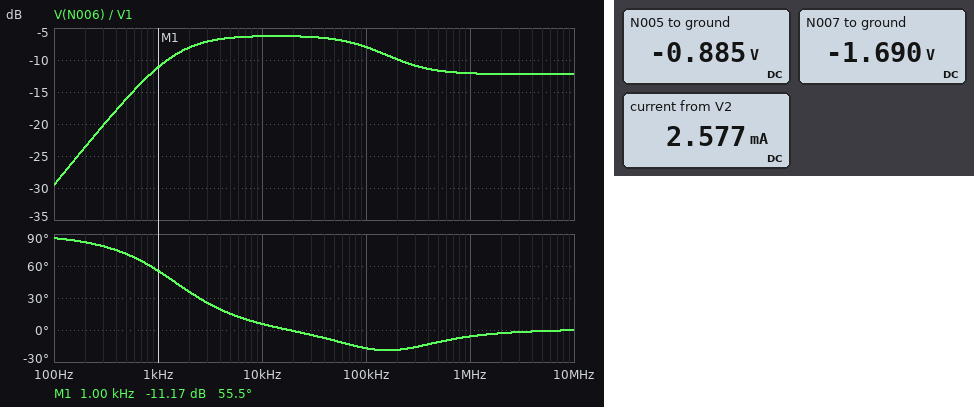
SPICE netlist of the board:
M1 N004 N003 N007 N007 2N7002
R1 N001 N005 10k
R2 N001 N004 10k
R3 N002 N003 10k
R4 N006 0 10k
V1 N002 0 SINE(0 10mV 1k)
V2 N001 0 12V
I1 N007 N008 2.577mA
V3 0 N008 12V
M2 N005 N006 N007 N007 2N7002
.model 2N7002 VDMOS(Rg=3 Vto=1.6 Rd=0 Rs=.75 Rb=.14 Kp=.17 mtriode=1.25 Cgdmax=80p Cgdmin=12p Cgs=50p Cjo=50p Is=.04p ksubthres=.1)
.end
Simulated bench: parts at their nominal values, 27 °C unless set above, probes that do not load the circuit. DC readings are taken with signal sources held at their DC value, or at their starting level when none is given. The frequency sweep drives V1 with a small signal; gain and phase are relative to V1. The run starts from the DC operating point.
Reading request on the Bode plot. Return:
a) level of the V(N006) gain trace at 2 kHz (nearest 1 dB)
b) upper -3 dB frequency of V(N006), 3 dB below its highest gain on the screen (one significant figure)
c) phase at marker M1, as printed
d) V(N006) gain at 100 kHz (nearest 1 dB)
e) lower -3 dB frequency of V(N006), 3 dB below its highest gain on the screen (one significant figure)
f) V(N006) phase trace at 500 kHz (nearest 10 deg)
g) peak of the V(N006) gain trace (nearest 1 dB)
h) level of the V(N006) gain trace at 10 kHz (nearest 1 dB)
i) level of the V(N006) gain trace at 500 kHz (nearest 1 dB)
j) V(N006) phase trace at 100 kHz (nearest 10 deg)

-8 dB
200 kHz
55.5 deg
-8 dB
1 kHz
-10 deg
-6 dB
-6 dB
-12 dB
-20 deg
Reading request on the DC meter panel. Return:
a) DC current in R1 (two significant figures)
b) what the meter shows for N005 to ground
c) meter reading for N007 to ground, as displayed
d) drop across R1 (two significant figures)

1.3 mA
-0.885 V
-1.690 V
13 V
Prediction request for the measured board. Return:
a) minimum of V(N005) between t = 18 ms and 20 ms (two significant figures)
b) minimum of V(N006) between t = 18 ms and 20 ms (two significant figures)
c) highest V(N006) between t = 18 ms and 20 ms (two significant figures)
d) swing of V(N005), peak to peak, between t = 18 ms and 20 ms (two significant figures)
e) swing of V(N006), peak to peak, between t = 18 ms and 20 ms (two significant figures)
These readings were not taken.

-1.5 V
-2.8 mV
2.8 mV
1.2 V
5.5 mV
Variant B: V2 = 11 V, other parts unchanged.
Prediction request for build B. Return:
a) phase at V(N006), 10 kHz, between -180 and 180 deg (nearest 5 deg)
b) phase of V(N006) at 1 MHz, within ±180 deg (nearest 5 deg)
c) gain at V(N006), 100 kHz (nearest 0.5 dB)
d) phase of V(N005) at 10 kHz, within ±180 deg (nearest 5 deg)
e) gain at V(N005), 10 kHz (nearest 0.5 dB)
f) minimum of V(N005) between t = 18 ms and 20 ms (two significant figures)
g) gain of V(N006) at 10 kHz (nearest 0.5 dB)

125 deg
10 deg
-17.5 dB
40 deg
-25.5 dB
-1.9 V
-47.5 dB
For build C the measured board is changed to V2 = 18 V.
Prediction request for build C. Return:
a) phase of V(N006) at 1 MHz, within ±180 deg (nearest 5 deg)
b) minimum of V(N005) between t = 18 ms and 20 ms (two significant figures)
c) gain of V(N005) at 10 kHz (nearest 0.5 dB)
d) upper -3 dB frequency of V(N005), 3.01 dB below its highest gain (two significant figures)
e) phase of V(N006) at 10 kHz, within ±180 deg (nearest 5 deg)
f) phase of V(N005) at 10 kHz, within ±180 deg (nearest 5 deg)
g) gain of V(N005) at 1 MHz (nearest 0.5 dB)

-20 deg
4.4 V
31.5 dB
6.1 kHz
30 deg
-60 deg
-8.0 dB
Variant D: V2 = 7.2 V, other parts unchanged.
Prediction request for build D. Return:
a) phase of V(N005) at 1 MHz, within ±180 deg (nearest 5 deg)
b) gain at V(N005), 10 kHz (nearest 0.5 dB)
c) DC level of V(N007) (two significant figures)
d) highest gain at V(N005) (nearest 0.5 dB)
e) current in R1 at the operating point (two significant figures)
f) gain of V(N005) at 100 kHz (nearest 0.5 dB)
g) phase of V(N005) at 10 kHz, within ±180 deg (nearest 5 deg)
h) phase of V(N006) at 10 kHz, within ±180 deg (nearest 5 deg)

5 deg
-28.0 dB
-5.7 V
-12.0 dB
1.3 mA
-13.5 dB
80 deg
165 deg
